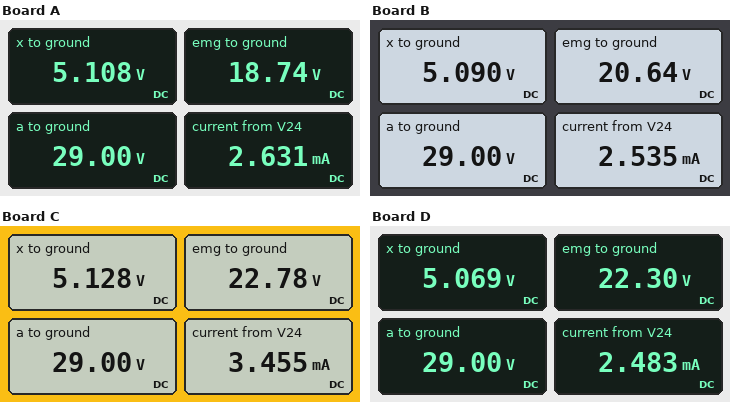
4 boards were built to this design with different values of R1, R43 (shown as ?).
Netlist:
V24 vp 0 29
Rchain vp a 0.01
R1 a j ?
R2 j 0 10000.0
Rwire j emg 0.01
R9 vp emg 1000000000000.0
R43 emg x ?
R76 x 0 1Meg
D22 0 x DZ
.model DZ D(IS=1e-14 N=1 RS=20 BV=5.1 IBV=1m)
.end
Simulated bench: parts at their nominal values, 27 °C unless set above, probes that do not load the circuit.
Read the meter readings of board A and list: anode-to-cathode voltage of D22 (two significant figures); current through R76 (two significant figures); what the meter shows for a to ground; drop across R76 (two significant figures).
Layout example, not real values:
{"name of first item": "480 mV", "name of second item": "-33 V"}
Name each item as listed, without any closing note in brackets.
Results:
{"anode-to-cathode voltage of D22": "-5.1 V", "current through R76": "5.1 µA", "what the meter shows for a to ground": "29.00 V", "drop across R76": "5.1 V"}
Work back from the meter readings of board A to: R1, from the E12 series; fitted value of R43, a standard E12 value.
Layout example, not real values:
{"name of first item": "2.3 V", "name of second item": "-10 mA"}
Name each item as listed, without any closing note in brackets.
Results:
{"R1, from the E12 series": "3.9 kΩ", "fitted value of R43, a standard E12 value": "18 kΩ"}
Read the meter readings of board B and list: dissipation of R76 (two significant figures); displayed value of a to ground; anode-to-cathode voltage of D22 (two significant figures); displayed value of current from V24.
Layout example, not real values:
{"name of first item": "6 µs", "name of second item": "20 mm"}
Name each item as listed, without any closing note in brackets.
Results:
{"dissipation of R76": "26 µW", "displayed value of a to ground": "29.00 V", "anode-to-cathode voltage of D22": "-5.1 V", "displayed value of current from V24": "2.535 mA"}
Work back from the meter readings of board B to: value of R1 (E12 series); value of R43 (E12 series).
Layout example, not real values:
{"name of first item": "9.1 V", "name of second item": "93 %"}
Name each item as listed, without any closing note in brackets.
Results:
{"value of R1": "3.3 kΩ", "value of R43": "33 kΩ"}
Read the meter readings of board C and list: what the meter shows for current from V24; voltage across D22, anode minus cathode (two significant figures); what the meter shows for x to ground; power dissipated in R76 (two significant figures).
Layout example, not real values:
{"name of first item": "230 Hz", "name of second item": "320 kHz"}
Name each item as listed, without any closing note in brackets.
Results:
{"what the meter shows for current from V24": "3.455 mA", "voltage across D22, anode minus cathode": "-5.1 V", "what the meter shows for x to ground": "5.128 V", "power dissipated in R76": "26 µW"}
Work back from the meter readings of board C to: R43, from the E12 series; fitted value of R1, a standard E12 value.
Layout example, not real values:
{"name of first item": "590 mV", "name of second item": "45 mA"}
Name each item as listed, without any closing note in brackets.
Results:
{"R43, from the E12 series": "15 kΩ", "fitted value of R1, a standard E12 value": "1.8 kΩ"}
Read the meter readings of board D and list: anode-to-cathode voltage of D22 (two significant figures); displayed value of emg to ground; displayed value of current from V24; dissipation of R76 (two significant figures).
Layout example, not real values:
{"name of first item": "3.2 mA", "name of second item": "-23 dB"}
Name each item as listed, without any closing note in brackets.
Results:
{"anode-to-cathode voltage of D22": "-5.1 V", "displayed value of emg to ground": "22.30 V", "displayed value of current from V24": "2.483 mA", "dissipation of R76": "26 µW"}
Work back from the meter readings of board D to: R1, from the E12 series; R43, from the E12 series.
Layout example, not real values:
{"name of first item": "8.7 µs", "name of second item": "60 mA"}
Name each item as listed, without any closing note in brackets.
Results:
{"R1, from the E12 series": "2.7 kΩ", "R43, from the E12 series": "68 kΩ"}
